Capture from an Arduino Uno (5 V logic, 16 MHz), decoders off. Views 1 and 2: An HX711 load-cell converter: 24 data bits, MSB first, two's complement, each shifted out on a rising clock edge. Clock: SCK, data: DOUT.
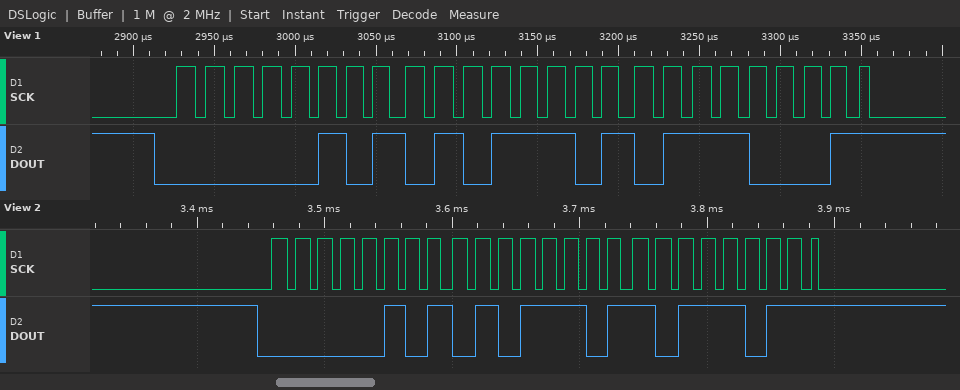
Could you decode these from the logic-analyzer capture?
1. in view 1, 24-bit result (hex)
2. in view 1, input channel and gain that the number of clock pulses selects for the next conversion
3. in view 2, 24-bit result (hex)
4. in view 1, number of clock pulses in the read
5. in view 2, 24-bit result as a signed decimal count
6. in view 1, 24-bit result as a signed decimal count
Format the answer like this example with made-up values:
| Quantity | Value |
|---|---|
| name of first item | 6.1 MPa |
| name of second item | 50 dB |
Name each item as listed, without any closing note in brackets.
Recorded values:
| Quantity | Value |
|---|---|
| in view 1, 24-bit result | 0x055D71 |
| in view 1, input channel and gain that the number of clock pulses selects for the next conversion | channel A, gain 128 |
| in view 2, 24-bit result | 0x055DBB |
| in view 1, number of clock pulses in the read | 25 |
| in view 2, 24-bit result as a signed decimal count | 351675 |
| in view 1, 24-bit result as a signed decimal count | 351601 |
